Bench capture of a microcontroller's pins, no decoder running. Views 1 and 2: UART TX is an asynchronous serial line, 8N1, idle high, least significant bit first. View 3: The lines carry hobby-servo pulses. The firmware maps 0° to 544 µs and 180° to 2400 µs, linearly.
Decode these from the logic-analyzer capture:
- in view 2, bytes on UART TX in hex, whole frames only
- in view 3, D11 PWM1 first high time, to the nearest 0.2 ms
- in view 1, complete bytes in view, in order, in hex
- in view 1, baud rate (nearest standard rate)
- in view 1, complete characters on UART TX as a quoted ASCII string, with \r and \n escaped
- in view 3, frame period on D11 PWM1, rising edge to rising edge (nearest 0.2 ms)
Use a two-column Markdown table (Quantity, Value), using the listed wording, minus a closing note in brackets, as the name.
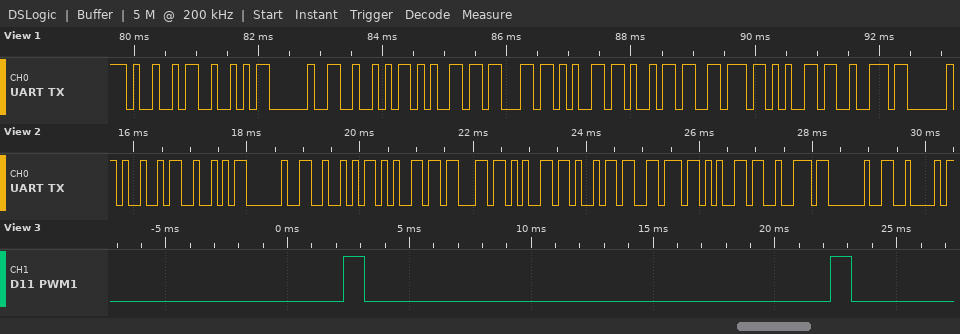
| Quantity | Value |
|---|---|
| in view 2, bytes on UART TX in hex, whole frames only | 49 52 20 52 65 63 65 69 76 65 72 20 42 |
| in view 3, D11 PWM1 first high time, to the nearest 0.2 ms | 0.8 ms |
| in view 1, complete bytes in view, in order, in hex | 0x49 0x52 0x20 0x52 0x65 0x63 0x65 0x69 0x76 0x65 0x72 |
| in view 1, baud rate | 9600 baud |
| in view 1, complete characters on UART TX as a quoted ASCII string, with \r and \n escaped | "IR Receiver" |
| in view 3, frame period on D11 PWM1, rising edge to rising edge | 20.0 ms |
